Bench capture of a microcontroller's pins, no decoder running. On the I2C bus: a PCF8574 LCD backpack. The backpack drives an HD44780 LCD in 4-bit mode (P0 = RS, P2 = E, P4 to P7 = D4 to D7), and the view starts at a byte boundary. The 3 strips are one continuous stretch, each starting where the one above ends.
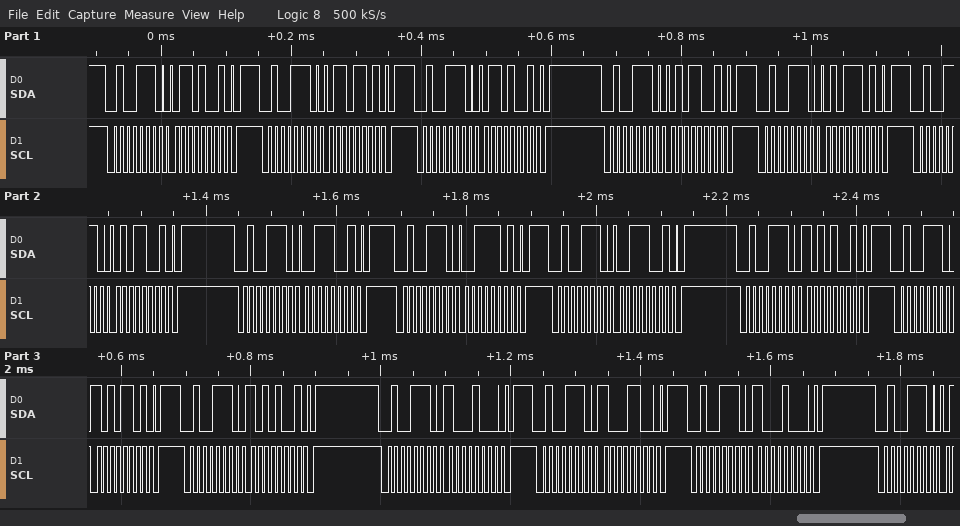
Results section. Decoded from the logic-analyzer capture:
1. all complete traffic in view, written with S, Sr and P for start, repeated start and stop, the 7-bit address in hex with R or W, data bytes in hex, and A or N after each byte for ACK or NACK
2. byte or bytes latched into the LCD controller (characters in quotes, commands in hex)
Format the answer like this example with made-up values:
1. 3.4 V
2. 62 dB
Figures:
1. S 27W A 69 A P S 27W A 6D A P S 27W A 69 A P S 27W A 59 A P S 27W A 5D A P S 27W A 59 A P S 27W A 39 A P S 27W A 3D A P S 27W A 39 A P S 27W A A9 A P S 27W A AD A P S 27W A A9 A P S 27W A 88 A P S 27W A 8C A P S 27W A 88 A P S 27W A
2. 'e' ':'
